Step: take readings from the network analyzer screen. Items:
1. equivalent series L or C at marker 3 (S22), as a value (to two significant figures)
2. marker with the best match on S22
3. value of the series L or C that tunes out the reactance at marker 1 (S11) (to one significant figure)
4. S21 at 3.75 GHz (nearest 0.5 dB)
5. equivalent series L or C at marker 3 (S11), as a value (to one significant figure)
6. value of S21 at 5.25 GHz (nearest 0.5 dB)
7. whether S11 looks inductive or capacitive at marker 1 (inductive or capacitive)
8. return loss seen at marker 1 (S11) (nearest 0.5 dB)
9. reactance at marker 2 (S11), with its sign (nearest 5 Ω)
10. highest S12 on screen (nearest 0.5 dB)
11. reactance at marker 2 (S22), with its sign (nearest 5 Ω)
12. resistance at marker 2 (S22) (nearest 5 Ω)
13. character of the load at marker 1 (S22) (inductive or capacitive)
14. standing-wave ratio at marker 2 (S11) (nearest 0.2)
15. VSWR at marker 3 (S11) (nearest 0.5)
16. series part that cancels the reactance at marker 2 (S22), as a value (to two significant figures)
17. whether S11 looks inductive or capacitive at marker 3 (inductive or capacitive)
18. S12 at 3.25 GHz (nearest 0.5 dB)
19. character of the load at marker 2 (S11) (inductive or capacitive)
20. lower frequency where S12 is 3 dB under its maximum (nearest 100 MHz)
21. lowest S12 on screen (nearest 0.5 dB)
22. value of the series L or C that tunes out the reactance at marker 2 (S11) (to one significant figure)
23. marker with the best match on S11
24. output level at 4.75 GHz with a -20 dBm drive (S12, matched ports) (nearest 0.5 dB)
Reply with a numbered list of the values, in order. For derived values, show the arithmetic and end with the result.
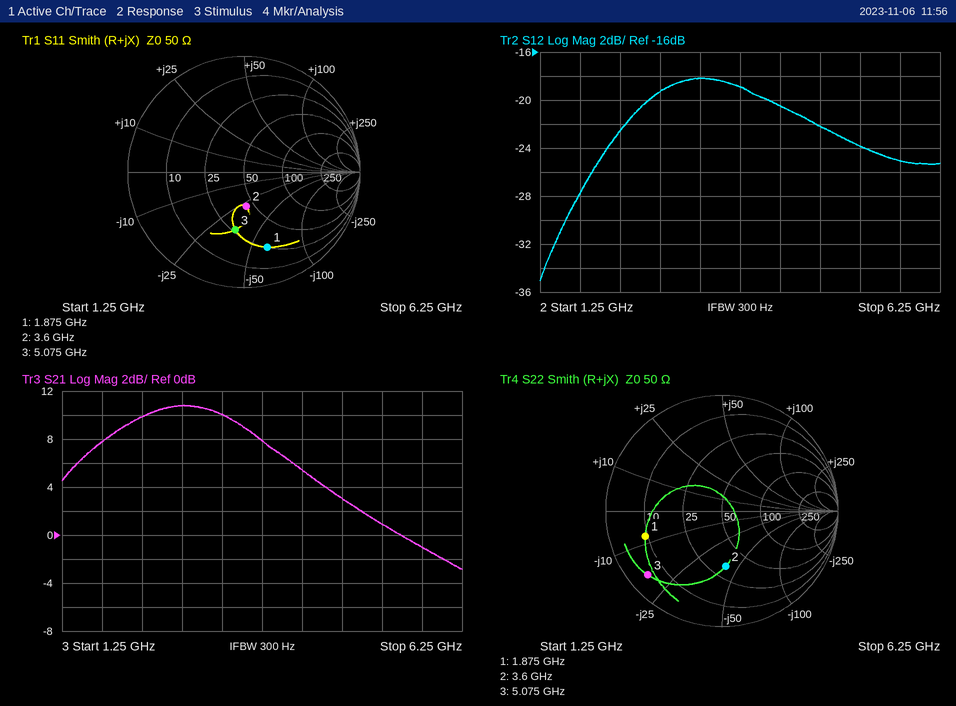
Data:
1. C = 1/(2π × 5.075 GHz × 18 Ω) ≈ 1.7 pF
2. marker 2
3. L = 60 Ω/(2π × 1.875 GHz) ≈ 5 nH
4. 8.0 dB
5. C = 1/(2π × 5.075 GHz × 35 Ω) ≈ 896 fF, so 900 fF to one significant figure
6. 1.0 dB
7. capacitive
8. 3.5 dB
9. -30 Ω
10. -18.0 dB
11. -40 Ω
12. 35 Ω
13. capacitive
14. 1.8
15. 3.0
16. L = 40 Ω/(2π × 3.6 GHz) ≈ 1.8 nH
17. capacitive
18. -18.0 dB
19. capacitive
20. 2.4 GHz
21. -35.0 dB
22. L = 30 Ω/(2π × 3.6 GHz) ≈ 1 nH
23. marker 2
24. -20 dBm + (-22.0 dB) = -42.0 dBm
